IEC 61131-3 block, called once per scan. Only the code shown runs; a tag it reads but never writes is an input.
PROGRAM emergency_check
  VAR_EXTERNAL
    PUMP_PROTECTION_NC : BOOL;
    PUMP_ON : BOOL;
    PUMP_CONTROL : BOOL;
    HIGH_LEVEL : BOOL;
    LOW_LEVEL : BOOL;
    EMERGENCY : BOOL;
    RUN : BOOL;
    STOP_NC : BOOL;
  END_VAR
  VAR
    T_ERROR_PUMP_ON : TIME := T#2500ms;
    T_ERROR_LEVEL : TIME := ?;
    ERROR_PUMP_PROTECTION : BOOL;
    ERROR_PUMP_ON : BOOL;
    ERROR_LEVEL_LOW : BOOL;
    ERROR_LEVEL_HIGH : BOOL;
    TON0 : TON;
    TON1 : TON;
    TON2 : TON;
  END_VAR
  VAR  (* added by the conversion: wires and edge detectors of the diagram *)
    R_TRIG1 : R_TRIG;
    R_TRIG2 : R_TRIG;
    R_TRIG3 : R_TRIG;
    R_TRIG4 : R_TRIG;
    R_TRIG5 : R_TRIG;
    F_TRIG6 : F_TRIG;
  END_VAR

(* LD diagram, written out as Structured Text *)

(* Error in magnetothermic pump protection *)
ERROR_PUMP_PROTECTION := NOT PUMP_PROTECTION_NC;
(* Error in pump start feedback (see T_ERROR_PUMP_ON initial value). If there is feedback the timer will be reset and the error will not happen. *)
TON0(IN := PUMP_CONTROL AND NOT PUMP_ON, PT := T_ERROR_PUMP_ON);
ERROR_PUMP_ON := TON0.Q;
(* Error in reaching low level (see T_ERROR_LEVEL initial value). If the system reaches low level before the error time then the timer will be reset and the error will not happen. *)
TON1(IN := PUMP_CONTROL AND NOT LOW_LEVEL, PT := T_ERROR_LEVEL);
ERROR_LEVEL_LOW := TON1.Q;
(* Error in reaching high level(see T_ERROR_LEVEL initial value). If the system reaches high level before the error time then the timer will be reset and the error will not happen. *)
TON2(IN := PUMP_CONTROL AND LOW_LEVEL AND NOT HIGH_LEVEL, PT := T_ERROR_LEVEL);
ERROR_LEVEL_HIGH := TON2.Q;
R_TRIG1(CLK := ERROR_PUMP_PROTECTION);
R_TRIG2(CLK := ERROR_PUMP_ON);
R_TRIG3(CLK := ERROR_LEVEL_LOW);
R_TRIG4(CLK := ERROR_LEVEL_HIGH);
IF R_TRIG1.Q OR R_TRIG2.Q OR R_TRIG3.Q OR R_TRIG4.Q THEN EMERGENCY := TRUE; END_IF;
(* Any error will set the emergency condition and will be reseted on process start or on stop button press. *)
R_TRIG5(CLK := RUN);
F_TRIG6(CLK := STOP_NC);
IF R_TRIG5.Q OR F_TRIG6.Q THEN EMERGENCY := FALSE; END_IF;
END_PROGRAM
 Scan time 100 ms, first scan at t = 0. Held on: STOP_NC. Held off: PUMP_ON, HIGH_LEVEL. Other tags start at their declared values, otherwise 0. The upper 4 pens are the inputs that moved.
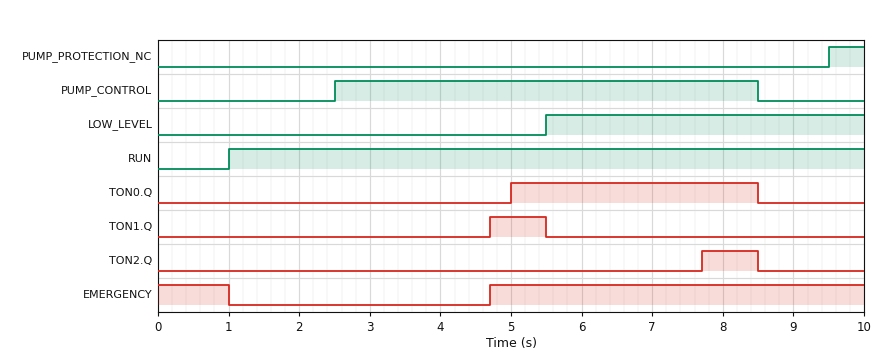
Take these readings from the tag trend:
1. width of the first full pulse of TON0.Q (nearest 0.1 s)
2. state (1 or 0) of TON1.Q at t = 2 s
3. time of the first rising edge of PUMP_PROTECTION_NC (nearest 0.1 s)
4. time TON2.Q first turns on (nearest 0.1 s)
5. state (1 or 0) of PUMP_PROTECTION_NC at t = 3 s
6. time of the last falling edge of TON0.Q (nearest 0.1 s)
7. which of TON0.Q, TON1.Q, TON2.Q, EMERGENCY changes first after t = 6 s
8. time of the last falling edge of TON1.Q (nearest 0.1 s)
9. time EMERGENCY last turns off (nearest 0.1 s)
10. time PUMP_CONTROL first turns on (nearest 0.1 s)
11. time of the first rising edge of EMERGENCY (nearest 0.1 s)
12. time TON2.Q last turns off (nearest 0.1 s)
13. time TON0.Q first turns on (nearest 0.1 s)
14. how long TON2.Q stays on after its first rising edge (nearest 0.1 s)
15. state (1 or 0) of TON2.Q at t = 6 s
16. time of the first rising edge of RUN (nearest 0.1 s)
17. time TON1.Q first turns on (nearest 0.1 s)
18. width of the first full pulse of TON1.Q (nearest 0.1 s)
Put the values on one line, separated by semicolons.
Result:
3.5 s; 0; 9.5 s; 7.7 s; 0; 8.5 s; TON2.Q; 5.5 s; 1.0 s; 2.5 s; 4.7 s; 8.5 s; 5.0 s; 0.8 s; 0; 1.0 s; 4.7 s; 0.8 s
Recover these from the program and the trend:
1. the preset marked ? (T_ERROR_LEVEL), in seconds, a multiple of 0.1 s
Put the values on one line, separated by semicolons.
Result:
2.2 s
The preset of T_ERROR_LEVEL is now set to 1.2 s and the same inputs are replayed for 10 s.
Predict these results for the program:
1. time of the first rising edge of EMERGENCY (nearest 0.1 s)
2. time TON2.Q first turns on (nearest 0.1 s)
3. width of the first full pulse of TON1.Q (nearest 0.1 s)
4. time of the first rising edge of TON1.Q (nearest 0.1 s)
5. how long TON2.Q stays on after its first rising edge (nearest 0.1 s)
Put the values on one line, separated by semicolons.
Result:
3.7 s; 6.7 s; 1.8 s; 3.7 s; 1.8 s
